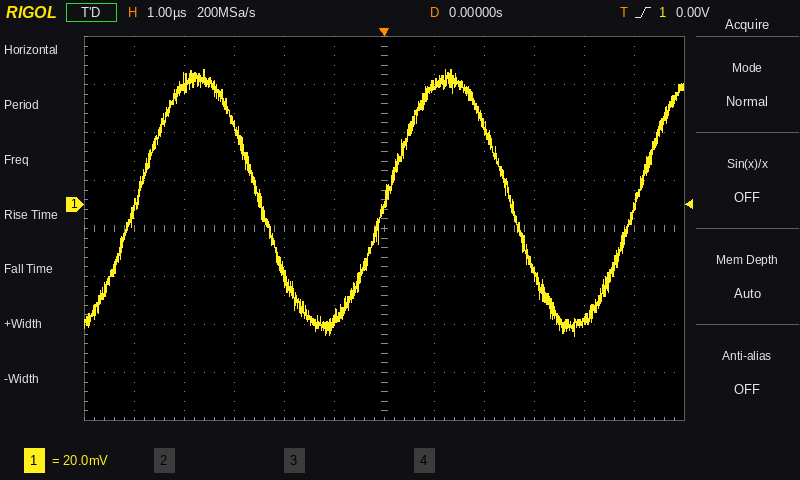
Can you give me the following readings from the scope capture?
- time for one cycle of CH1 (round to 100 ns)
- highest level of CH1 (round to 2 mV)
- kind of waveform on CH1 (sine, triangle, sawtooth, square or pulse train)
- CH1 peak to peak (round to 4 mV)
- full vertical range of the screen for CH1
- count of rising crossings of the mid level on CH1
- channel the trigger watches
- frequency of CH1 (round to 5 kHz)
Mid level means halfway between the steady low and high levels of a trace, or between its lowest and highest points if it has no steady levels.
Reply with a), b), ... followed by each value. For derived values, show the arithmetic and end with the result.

a) 5.0 µs
b) 56 mV
c) sine
d) 112 mV
e) 160 mV
f) 3
g) CH1
h) 1 / 5.0 µs ≈ 200 kHz
